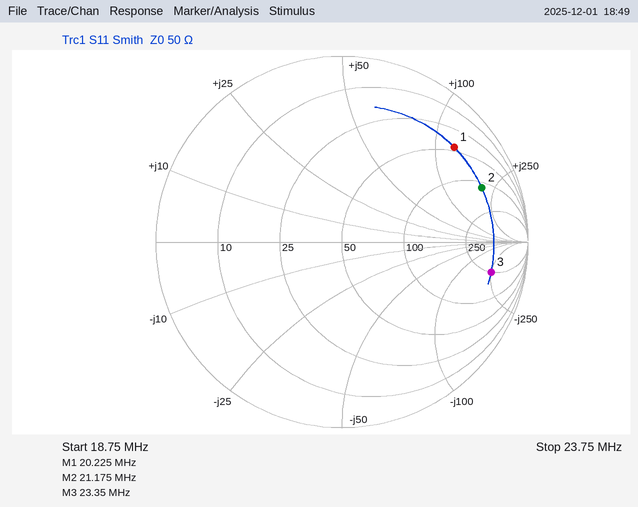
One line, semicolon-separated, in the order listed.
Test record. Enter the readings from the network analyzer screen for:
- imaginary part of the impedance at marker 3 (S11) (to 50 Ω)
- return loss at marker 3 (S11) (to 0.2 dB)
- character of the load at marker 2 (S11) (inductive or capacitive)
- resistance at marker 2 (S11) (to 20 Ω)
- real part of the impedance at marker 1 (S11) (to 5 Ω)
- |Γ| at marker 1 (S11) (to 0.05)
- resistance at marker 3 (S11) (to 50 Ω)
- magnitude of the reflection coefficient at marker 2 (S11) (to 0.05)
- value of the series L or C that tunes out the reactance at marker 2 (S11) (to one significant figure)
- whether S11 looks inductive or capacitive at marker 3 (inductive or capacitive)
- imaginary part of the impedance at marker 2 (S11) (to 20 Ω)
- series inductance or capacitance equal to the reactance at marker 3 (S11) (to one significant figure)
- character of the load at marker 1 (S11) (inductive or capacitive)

-250 Ω; 1.8 dB; inductive; 120 Ω; 45 Ω; 0.80; 250 Ω; 0.80; 40 pF; capacitive; +200 Ω; 30 pF; inductive
